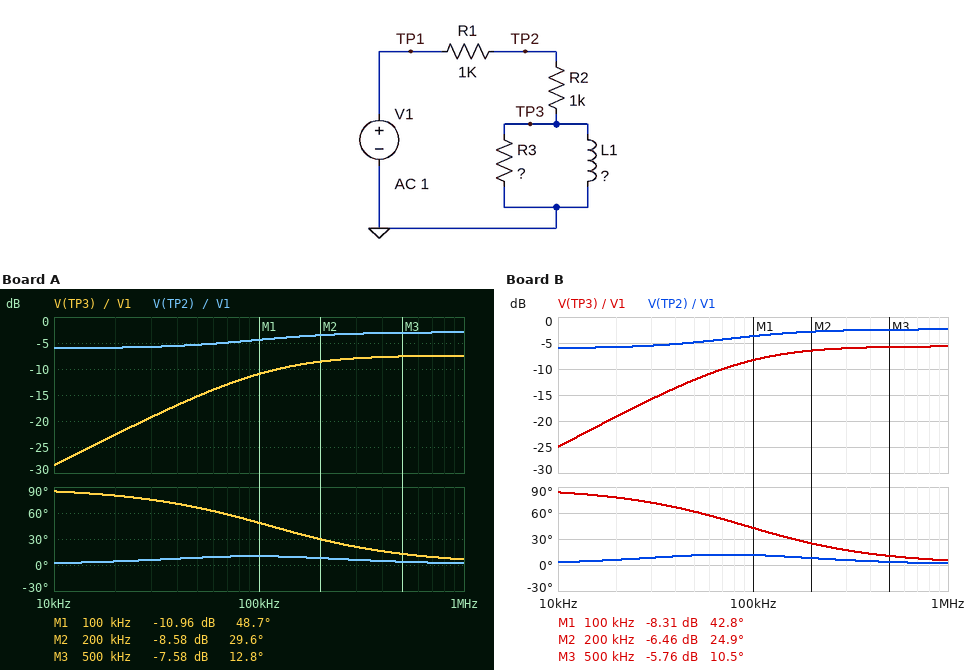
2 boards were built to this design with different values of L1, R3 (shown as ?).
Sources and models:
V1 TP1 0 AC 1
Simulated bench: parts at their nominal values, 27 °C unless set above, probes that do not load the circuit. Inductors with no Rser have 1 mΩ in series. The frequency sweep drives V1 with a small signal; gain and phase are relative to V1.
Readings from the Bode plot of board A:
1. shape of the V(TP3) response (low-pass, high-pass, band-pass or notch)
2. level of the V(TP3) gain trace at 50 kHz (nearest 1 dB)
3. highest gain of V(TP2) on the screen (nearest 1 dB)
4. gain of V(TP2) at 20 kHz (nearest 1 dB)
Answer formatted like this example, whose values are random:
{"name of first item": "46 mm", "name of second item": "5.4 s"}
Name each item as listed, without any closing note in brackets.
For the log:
{"shape of the V(TP3) response": "high-pass", "level of the V(TP3) gain trace at 50 kHz": "-15 dB", "highest gain of V(TP2) on the screen": "-3 dB", "gain of V(TP2) at 20 kHz": "-6 dB"}
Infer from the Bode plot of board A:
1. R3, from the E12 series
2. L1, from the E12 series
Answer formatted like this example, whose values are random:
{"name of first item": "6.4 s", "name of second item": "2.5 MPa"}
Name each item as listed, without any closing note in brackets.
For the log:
{"R3, from the E12 series": "1.5 kΩ", "L1, from the E12 series": "1.2 mH"}
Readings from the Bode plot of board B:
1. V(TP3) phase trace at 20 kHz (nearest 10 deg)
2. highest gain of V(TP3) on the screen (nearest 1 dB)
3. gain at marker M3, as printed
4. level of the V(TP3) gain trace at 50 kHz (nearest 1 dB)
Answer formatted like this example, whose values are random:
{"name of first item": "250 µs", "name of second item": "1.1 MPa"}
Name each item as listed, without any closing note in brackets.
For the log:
{"V(TP3) phase trace at 20 kHz": "80 deg", "highest gain of V(TP3) on the screen": "-6 dB", "gain at marker M3, as printed": "-5.76 dB", "level of the V(TP3) gain trace at 50 kHz": "-12 dB"}
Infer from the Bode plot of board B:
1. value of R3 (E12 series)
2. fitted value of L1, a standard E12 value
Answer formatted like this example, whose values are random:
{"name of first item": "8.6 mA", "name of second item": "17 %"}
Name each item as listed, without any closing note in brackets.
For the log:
{"value of R3": "2.2 kΩ", "fitted value of L1, a standard E12 value": "1.8 mH"}
